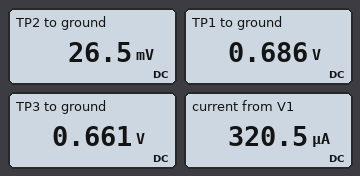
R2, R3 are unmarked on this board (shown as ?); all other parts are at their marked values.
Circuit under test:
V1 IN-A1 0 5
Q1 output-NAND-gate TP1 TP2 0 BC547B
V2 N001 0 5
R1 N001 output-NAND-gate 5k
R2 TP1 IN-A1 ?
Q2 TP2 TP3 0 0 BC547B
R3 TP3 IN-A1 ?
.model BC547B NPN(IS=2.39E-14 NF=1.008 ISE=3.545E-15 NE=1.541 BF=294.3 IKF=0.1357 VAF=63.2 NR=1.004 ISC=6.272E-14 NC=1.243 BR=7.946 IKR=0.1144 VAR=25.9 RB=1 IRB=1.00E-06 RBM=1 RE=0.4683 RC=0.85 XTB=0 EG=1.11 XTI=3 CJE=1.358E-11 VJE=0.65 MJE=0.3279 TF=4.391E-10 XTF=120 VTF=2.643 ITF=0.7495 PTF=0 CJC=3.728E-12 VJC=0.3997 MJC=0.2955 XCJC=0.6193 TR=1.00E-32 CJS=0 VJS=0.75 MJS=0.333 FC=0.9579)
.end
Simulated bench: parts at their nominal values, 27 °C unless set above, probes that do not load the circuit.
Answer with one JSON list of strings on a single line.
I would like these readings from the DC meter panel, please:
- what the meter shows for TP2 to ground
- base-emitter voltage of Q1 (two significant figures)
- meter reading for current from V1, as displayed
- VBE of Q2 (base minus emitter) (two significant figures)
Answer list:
["26.5 mV", "660 mV", "320.5 µA", "660 mV"]
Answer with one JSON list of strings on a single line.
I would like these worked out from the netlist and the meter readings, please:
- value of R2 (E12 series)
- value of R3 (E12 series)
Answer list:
["27 kΩ", "27 kΩ"]
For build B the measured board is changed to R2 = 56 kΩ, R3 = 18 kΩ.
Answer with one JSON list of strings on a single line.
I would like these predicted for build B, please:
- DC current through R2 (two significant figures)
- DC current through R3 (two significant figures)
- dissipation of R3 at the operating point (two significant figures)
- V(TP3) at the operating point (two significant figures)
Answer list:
["77 µA", "240 µA", "1.0 mW", "670 mV"]
